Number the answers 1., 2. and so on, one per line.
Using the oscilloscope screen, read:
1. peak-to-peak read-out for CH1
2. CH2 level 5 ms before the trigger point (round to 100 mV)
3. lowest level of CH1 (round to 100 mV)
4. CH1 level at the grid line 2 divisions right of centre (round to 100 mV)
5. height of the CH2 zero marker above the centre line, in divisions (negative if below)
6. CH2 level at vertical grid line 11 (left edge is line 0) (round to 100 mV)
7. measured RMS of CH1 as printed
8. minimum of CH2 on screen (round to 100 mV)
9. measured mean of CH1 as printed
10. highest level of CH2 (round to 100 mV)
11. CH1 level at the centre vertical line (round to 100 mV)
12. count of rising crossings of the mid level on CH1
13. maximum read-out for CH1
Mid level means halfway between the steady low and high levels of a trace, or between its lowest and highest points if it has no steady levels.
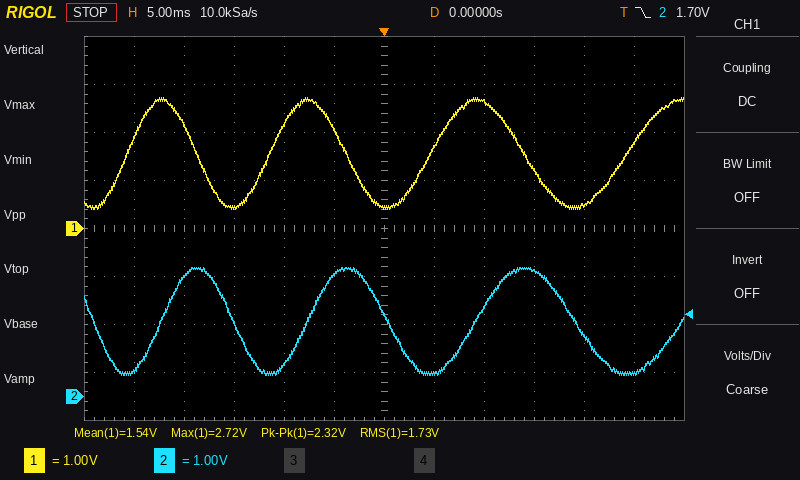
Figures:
1. 2.32 V
2. 2.5 V
3. 400 mV
4. 2.6 V
5. -3.5 div
6. 500 mV
7. 1.73 V
8. 400 mV
9. 1.54 V
10. 2.7 V
11. 400 mV
12. 4
13. 2.72 V
